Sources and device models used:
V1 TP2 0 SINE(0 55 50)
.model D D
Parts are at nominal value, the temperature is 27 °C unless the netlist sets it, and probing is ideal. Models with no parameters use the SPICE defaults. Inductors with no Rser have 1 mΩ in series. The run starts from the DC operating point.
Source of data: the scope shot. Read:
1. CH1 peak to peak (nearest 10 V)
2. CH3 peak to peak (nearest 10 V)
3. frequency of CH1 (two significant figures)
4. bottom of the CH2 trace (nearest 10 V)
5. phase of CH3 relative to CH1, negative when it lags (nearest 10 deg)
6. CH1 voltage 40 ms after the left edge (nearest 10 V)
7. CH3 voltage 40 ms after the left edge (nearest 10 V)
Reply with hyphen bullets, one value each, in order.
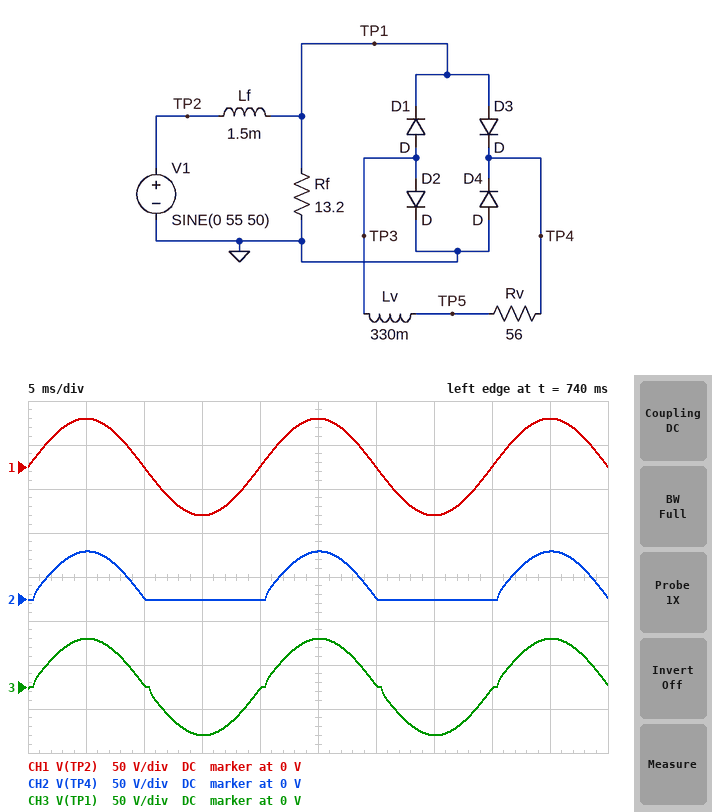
- 110 V
- 110 V
- 50 Hz
- 0 V
- 0 deg
- 0 V
- 0 V
